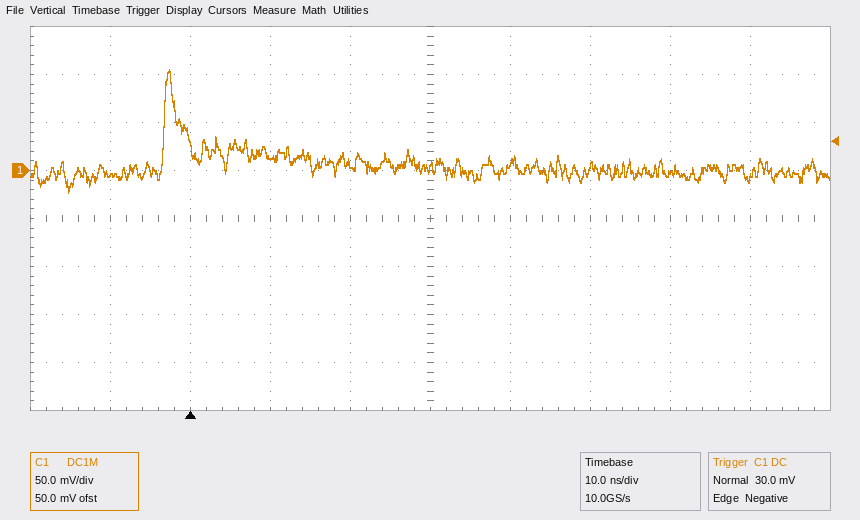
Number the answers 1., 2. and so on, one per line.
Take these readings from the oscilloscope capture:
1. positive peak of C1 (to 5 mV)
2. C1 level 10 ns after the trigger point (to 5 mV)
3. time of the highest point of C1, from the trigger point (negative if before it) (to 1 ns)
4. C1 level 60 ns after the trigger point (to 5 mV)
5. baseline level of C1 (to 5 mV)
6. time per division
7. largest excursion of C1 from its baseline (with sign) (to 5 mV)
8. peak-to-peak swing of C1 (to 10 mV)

1. 105 mV
2. 15 mV
3. -3 ns
4. -5 mV
5. 0 mV
6. 10 ns
7. +105 mV
8. 130 mV
